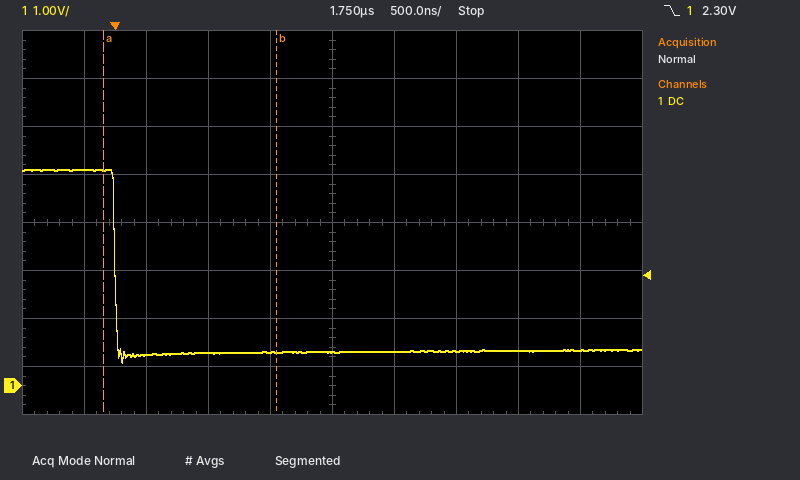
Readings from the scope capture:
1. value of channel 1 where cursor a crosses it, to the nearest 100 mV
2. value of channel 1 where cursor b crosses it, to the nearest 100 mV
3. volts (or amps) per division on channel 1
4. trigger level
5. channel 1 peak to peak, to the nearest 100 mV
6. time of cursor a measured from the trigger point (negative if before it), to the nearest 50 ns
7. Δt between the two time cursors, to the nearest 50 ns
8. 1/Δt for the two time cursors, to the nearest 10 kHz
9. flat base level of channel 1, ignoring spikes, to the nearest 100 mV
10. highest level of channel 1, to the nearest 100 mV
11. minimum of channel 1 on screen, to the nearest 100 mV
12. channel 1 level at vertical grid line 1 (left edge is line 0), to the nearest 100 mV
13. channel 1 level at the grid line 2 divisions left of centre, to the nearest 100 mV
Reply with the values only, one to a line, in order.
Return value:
4.5 V
700 mV
1 V
2.30 V
4.0 V
-100 ns
1.40 µs
710 kHz
700 mV
4.5 V
500 mV
4.5 V
700 mV
